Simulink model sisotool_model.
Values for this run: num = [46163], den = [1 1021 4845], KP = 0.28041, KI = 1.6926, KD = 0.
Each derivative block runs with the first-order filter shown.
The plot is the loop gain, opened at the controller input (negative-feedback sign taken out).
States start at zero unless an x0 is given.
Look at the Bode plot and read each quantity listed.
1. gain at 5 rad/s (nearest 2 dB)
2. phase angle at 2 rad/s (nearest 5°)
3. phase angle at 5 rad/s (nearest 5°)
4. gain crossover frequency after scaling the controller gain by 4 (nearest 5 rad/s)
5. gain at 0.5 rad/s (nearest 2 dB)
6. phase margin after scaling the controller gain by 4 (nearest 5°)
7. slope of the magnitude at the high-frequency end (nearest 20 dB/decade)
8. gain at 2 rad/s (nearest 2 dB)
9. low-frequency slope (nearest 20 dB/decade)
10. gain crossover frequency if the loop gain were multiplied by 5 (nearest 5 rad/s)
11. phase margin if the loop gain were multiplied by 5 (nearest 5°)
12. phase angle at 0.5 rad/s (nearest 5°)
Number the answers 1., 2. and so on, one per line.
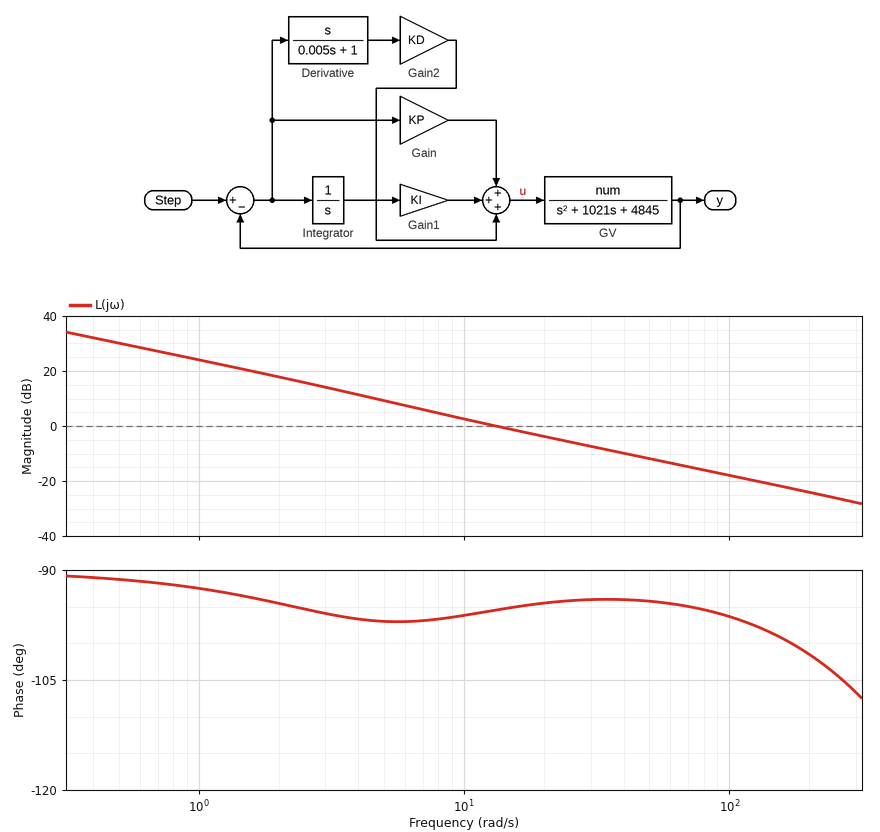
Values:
1. 10 dB
2. -95°
3. -95°
4. 50 rad/s
5. 30 dB
6. 85°
7. -20 dB/decade
8. 18 dB
9. -20 dB/decade
10. 65 rad/s
11. 85°
12. -90°
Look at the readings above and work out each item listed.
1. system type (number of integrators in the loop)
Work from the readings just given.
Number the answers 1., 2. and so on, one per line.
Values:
1. 1
